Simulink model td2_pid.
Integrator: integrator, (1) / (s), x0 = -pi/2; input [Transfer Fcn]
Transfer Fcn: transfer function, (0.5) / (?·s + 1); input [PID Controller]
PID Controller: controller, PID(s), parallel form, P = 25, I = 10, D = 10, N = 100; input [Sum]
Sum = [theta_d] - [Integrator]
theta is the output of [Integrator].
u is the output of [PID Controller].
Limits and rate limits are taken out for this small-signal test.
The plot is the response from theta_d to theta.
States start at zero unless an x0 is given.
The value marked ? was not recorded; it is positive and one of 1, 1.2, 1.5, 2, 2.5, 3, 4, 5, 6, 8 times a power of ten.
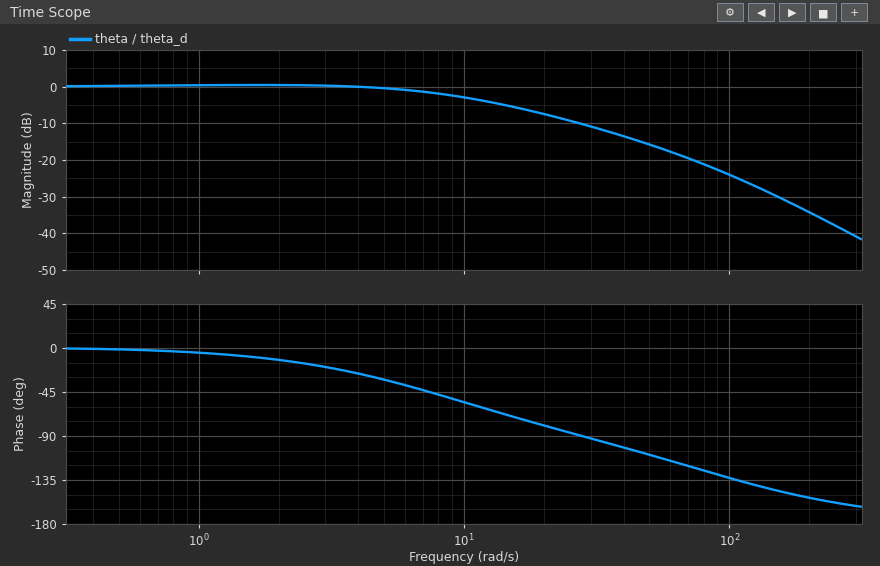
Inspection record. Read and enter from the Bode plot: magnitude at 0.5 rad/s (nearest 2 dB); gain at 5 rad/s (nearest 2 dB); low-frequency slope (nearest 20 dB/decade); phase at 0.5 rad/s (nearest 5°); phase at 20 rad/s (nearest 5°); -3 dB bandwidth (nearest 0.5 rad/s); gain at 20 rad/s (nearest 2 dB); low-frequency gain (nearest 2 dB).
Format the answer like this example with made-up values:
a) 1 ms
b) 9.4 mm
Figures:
a) 0 dB
b) 0 dB
c) 0 dB/decade
d) 0°
e) -80°
f) 10.0 rad/s
g) -8 dB
h) 0 dB
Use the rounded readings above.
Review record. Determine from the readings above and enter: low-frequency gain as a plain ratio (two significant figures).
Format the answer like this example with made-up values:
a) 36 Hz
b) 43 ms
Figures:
a) 1.0
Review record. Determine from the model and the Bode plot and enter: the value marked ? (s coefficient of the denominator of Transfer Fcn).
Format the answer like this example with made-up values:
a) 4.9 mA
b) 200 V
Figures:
a) 0.6
